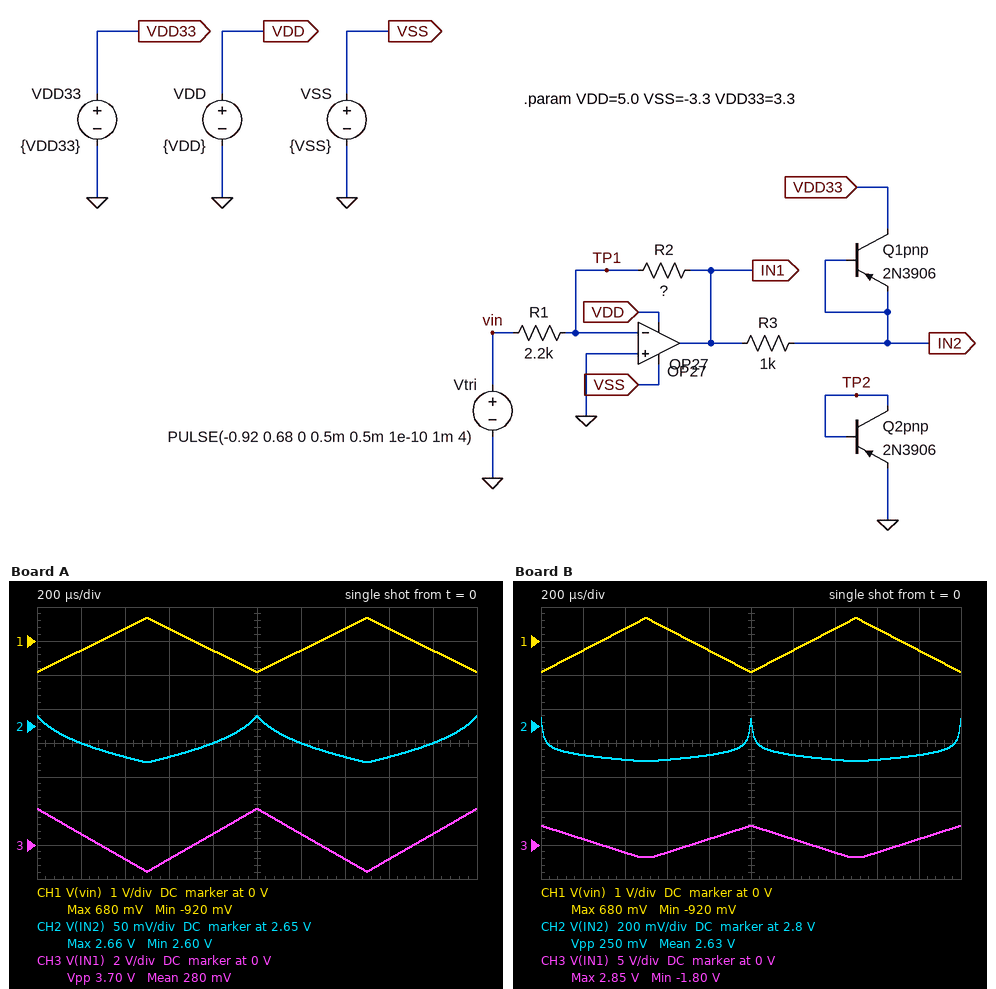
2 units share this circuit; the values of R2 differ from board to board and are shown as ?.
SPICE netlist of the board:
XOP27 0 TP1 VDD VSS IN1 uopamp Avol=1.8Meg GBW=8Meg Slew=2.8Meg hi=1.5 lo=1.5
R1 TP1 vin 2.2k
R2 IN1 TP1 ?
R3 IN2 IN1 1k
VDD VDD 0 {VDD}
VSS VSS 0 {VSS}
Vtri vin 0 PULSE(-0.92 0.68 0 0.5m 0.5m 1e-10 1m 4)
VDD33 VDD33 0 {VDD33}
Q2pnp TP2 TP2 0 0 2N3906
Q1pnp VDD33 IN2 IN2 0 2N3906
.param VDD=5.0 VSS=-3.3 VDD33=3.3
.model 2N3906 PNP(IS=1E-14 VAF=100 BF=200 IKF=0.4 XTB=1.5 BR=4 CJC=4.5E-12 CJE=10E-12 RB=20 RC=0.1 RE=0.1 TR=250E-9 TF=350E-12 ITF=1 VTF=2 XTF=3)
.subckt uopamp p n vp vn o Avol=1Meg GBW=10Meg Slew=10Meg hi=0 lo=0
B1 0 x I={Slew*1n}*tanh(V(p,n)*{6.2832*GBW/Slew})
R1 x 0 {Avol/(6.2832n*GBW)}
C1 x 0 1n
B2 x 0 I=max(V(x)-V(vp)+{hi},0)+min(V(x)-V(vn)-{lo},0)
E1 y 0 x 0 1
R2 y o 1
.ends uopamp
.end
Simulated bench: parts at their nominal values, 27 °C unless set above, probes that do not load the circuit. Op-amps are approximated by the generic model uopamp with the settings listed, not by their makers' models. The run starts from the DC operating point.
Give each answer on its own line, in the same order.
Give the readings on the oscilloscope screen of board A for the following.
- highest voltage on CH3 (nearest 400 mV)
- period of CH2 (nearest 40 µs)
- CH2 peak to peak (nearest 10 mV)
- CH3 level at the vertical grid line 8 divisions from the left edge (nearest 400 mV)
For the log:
2.0 V
1.00 ms
70 mV
-800 mV
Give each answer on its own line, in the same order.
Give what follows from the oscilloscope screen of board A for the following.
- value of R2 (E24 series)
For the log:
5.1 kΩ
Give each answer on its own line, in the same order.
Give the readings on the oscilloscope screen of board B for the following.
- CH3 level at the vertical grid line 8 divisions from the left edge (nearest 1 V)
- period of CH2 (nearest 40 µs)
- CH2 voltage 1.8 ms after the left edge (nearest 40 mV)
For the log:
-1 V
1.00 ms
2.64 V
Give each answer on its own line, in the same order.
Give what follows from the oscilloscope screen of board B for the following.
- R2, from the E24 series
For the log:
6.8 kΩ
